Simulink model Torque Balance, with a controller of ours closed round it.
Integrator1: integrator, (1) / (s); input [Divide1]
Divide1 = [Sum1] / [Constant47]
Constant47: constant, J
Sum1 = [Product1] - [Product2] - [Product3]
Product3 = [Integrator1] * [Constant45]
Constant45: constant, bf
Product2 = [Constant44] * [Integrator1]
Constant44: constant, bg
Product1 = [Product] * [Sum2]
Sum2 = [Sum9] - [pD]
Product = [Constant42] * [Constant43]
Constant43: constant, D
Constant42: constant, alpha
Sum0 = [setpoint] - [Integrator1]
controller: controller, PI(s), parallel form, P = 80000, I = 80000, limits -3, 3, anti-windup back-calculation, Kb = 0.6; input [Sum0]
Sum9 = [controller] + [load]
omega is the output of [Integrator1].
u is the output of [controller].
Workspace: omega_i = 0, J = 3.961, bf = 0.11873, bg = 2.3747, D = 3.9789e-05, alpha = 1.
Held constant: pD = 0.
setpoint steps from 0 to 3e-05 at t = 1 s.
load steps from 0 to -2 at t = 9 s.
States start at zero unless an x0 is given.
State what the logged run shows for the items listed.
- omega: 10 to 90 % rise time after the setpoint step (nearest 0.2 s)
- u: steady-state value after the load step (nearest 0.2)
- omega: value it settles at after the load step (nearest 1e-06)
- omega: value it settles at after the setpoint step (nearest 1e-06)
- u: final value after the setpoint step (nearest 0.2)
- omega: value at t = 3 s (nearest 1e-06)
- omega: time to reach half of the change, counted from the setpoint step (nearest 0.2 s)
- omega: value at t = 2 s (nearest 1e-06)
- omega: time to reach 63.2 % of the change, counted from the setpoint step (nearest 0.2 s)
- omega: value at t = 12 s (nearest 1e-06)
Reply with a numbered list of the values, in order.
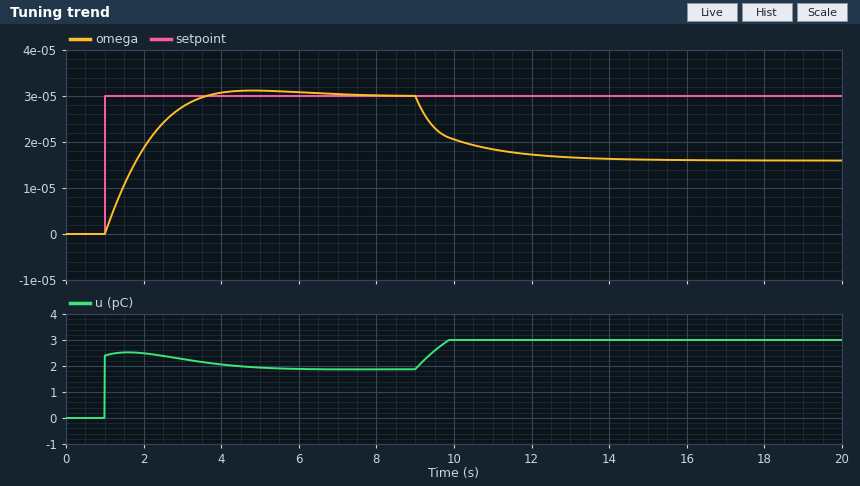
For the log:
1. 1.8 s
2. 3.0
3. 0.000016
4. 0.000030
5. 1.8
6. 0.000028
7. 0.8 s
8. 0.000019
9. 1.0 s
10. 0.000017
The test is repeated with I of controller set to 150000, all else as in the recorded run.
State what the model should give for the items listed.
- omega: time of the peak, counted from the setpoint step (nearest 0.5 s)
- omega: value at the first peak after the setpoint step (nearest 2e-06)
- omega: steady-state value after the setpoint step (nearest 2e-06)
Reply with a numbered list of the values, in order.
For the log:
1. 2.5 s
2. 0.000034
3. 0.000030
